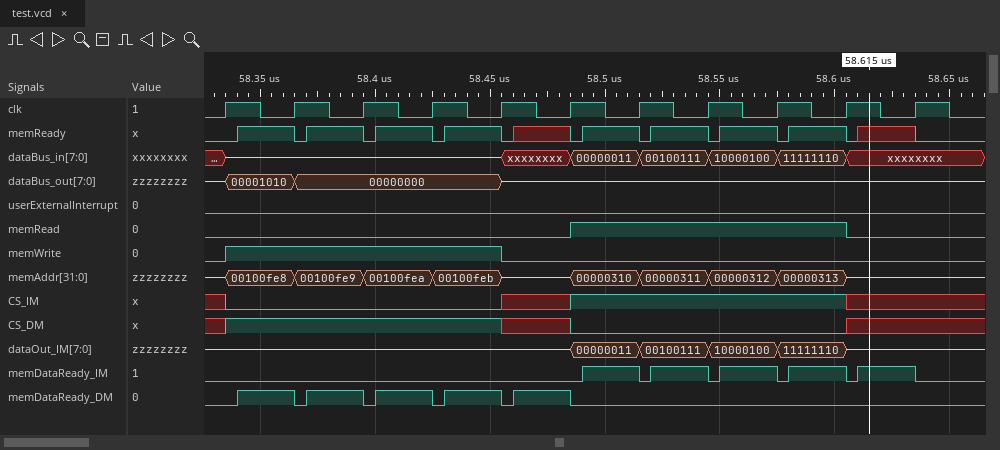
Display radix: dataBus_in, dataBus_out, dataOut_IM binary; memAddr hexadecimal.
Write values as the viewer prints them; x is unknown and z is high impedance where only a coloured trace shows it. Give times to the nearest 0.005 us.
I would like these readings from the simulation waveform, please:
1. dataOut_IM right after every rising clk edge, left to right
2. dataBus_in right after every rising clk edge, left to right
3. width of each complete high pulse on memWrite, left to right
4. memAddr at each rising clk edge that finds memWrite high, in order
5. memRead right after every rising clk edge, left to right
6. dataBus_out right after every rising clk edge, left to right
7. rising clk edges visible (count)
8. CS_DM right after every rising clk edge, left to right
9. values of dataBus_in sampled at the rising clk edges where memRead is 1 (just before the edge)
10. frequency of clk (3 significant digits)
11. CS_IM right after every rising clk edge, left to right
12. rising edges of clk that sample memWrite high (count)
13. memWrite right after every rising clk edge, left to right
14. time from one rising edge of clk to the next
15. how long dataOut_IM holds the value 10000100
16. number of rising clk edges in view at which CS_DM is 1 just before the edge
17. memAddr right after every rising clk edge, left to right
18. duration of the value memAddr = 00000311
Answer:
z, z, z, z, z, 00000011, 00100111, 10000100, 11111110, z, z
z, z, z, z, xxxxxxxx, 00000011, 00100111, 10000100, 11111110, xxxxxxxx, xxxxxxxx
0.12 us
00100fe8, 00100fe9, 00100fea, 00100feb
0 0 0 0 0 1 1 1 1 0 0
00001010, 00000000, 00000000, 00000000, z, z, z, z, z, z, z
11
1 1 1 1 x 0 0 0 0 x x
00000011, 00100111, 10000100, 11111110
33.3 MHz
0 0 0 0 x 1 1 1 1 x x
4
1 1 1 1 0 0 0 0 0 0 0
0.03 us
0.03 us
4
00100fe8, 00100fe9, 00100fea, 00100feb, z, 00000310, 00000311, 00000312, 00000313, z, z
0.03 us
